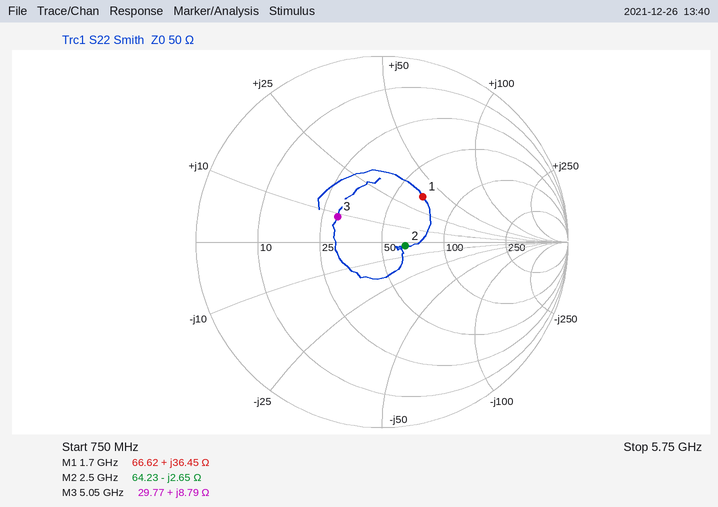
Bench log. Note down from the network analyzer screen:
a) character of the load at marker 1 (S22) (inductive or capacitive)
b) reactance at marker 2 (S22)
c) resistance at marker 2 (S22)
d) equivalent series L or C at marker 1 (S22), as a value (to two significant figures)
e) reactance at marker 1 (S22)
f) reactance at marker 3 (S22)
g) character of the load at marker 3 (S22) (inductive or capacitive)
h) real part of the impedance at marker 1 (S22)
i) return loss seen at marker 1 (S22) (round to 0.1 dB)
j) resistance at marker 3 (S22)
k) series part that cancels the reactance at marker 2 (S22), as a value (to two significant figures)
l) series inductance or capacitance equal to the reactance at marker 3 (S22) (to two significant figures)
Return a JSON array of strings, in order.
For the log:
["inductive", "-2.65 Ω", "64.23 Ω", "3.4 nH", "+36.45 Ω", "+8.79 Ω", "inductive", "66.62 Ω", "9.7 dB", "29.77 Ω", "170 pH", "280 pH"]
